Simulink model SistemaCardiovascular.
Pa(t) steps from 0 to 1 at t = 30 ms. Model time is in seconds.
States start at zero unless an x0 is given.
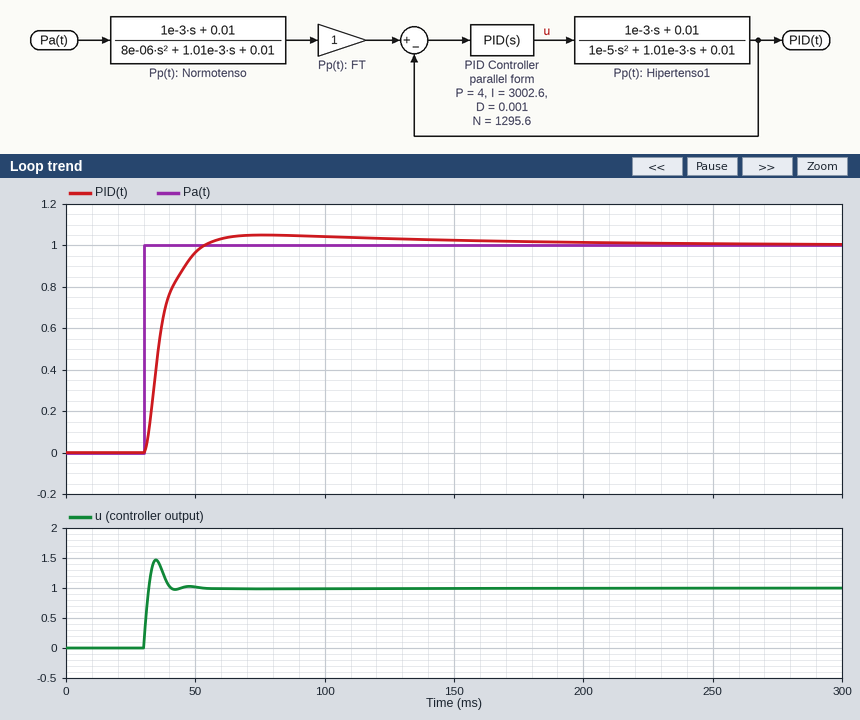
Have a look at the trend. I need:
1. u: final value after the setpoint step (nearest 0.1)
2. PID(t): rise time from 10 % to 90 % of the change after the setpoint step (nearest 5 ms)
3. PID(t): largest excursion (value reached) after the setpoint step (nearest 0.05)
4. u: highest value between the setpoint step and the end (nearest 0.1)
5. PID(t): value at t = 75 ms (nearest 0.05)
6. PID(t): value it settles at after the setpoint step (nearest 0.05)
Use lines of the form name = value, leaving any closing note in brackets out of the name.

u: final value after the setpoint step = 1.0
PID(t): rise time from 10 % to 90 % of the change after the setpoint step = 15 ms
PID(t): largest excursion (value reached) after the setpoint step = 1.05
u: highest value between the setpoint step and the end = 1.5
PID(t): value at t = 75 ms = 1.05
PID(t): value it settles at after the setpoint step = 1.00
